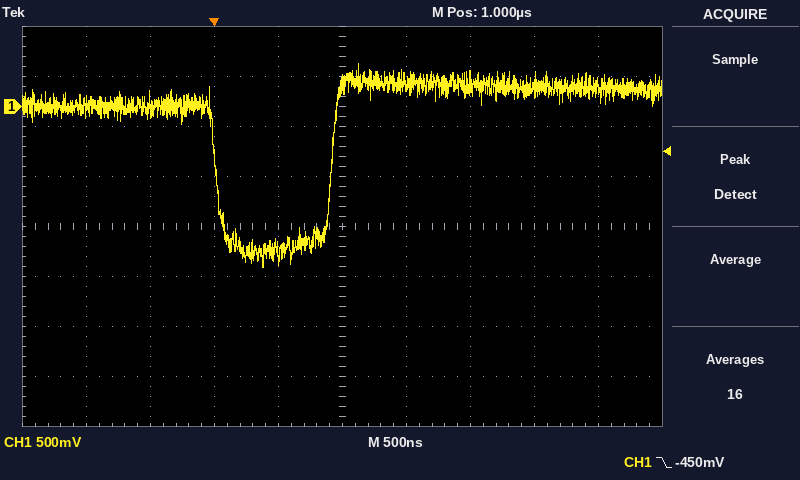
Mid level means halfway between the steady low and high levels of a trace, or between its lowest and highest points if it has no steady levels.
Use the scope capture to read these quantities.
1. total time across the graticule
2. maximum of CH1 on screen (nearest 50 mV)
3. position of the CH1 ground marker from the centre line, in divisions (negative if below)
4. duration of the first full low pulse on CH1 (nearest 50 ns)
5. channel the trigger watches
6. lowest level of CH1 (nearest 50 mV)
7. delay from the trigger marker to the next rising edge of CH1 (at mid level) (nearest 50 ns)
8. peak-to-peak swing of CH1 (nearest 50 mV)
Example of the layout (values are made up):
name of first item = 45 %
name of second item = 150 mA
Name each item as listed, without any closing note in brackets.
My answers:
total time across the graticule = 5 µs
maximum of CH1 on screen = 450 mV
position of the CH1 ground marker from the centre line, in divisions = +2.4 div
duration of the first full low pulse on CH1 = 900 ns
channel the trigger watches = CH1
lowest level of CH1 = -1.60 V
delay from the trigger marker to the next rising edge of CH1 (at mid level) = 900 ns
peak-to-peak swing of CH1 = 2.05 V
